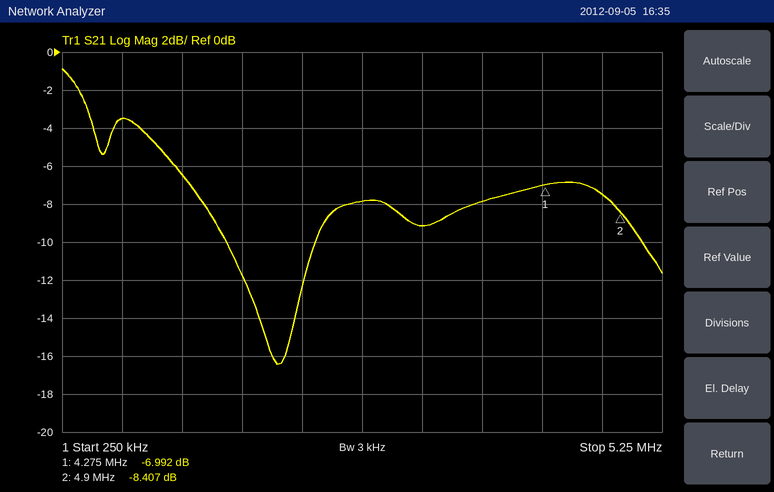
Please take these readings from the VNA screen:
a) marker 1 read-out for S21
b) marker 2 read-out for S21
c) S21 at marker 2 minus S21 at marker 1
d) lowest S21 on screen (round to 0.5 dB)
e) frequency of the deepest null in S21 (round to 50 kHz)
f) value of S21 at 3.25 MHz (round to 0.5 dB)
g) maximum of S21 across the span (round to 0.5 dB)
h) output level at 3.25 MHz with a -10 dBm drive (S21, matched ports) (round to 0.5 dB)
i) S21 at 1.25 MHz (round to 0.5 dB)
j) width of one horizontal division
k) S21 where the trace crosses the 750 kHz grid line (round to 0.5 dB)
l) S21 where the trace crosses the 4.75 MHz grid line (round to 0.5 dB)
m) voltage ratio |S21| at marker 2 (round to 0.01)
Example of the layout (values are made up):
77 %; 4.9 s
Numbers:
-6.992 dB; -8.407 dB; -1.415 dB; -16.5 dB; 2.05 MHz; -9.0 dB; -1.0 dB; -19.0 dBm; -6.5 dB; 500 kHz; -3.5 dB; -7.5 dB; 0.38
